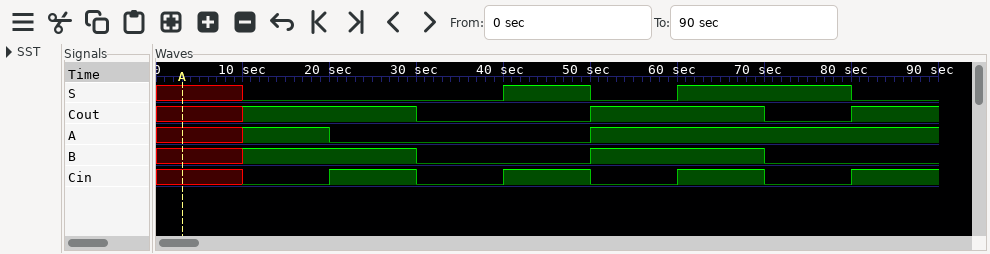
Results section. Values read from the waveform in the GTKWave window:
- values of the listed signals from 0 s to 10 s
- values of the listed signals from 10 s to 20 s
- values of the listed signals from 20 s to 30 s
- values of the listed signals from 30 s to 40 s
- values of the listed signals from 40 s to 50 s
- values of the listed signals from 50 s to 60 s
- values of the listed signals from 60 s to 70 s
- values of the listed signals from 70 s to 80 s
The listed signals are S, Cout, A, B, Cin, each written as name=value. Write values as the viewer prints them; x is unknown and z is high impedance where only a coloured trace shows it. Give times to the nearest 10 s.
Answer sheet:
S=x, Cout=x, A=x, B=x, Cin=x
S=0, Cout=1, A=1, B=1, Cin=0
S=0, Cout=1, A=0, B=1, Cin=1
S=0, Cout=0, A=0, B=0, Cin=0
S=1, Cout=0, A=0, B=0, Cin=1
S=0, Cout=1, A=1, B=1, Cin=0
S=1, Cout=1, A=1, B=1, Cin=1
S=1, Cout=0, A=1, B=0, Cin=0
